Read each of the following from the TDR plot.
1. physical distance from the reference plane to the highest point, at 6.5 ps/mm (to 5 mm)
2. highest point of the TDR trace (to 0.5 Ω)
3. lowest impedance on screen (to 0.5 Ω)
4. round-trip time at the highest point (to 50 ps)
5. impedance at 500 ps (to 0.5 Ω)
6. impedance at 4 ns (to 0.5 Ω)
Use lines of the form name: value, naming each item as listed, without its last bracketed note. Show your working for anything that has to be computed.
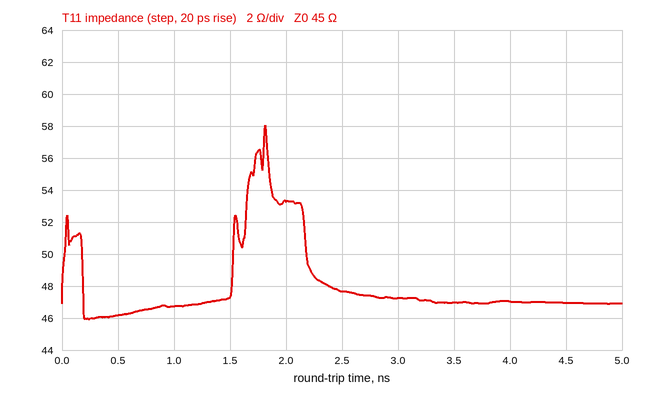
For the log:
physical distance from the reference plane to the highest point, at 6.5 ps/mm: 1.80 ns / 2 / 6.5 ps/mm ≈ 138 mm, so 140 mm to the nearest 5 mm
highest point of the TDR trace: 58.0 Ω
lowest impedance on screen: 46.0 Ω
round-trip time at the highest point: 1.80 ns
impedance at 500 ps: 46.0 Ω
impedance at 4 ns: 47.0 Ω
